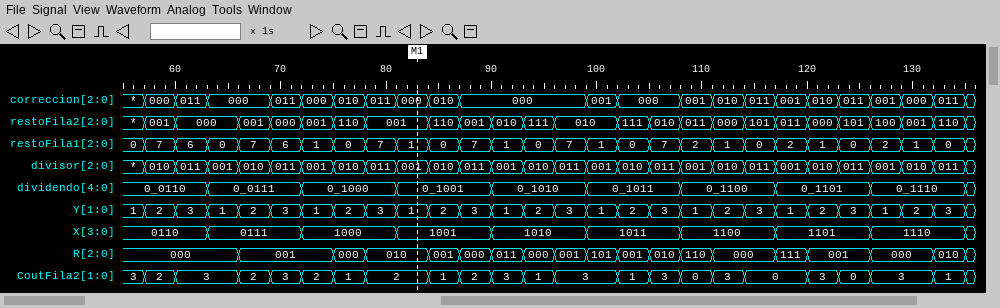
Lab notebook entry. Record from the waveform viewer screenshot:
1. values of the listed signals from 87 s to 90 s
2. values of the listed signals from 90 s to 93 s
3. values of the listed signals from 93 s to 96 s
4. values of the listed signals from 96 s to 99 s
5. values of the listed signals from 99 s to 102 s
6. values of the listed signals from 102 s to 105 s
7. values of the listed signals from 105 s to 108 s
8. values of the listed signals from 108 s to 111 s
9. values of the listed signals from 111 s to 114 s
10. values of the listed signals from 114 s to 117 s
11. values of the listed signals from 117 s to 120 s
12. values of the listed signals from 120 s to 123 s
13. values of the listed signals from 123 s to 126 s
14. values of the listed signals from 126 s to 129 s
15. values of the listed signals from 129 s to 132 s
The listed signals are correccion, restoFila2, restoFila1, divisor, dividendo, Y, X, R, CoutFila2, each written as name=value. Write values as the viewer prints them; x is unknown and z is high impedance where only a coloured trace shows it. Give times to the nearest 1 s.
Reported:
correccion=000, restoFila2=001, restoFila1=7, divisor=011, dividendo=0_1001, Y=3, X=1001, R=000, CoutFila2=2
correccion=000, restoFila2=010, restoFila1=1, divisor=001, dividendo=0_1010, Y=1, X=1010, R=011, CoutFila2=3
correccion=000, restoFila2=111, restoFila1=0, divisor=010, dividendo=0_1010, Y=2, X=1010, R=000, CoutFila2=1
correccion=000, restoFila2=010, restoFila1=7, divisor=011, dividendo=0_1010, Y=3, X=1010, R=001, CoutFila2=3
correccion=001, restoFila2=010, restoFila1=1, divisor=001, dividendo=0_1011, Y=1, X=1011, R=101, CoutFila2=3
correccion=000, restoFila2=111, restoFila1=0, divisor=010, dividendo=0_1011, Y=2, X=1011, R=001, CoutFila2=1
correccion=000, restoFila2=010, restoFila1=7, divisor=011, dividendo=0_1011, Y=3, X=1011, R=010, CoutFila2=3
correccion=001, restoFila2=011, restoFila1=2, divisor=001, dividendo=0_1100, Y=1, X=1100, R=110, CoutFila2=0
correccion=010, restoFila2=000, restoFila1=1, divisor=010, dividendo=0_1100, Y=2, X=1100, R=000, CoutFila2=3
correccion=011, restoFila2=101, restoFila1=0, divisor=011, dividendo=0_1100, Y=3, X=1100, R=000, CoutFila2=0
correccion=001, restoFila2=011, restoFila1=2, divisor=001, dividendo=0_1101, Y=1, X=1101, R=111, CoutFila2=0
correccion=010, restoFila2=000, restoFila1=1, divisor=010, dividendo=0_1101, Y=2, X=1101, R=001, CoutFila2=3
correccion=011, restoFila2=101, restoFila1=0, divisor=011, dividendo=0_1101, Y=3, X=1101, R=001, CoutFila2=0
correccion=001, restoFila2=100, restoFila1=2, divisor=001, dividendo=0_1110, Y=1, X=1110, R=000, CoutFila2=3
correccion=000, restoFila2=001, restoFila1=1, divisor=010, dividendo=0_1110, Y=2, X=1110, R=000, CoutFila2=3
